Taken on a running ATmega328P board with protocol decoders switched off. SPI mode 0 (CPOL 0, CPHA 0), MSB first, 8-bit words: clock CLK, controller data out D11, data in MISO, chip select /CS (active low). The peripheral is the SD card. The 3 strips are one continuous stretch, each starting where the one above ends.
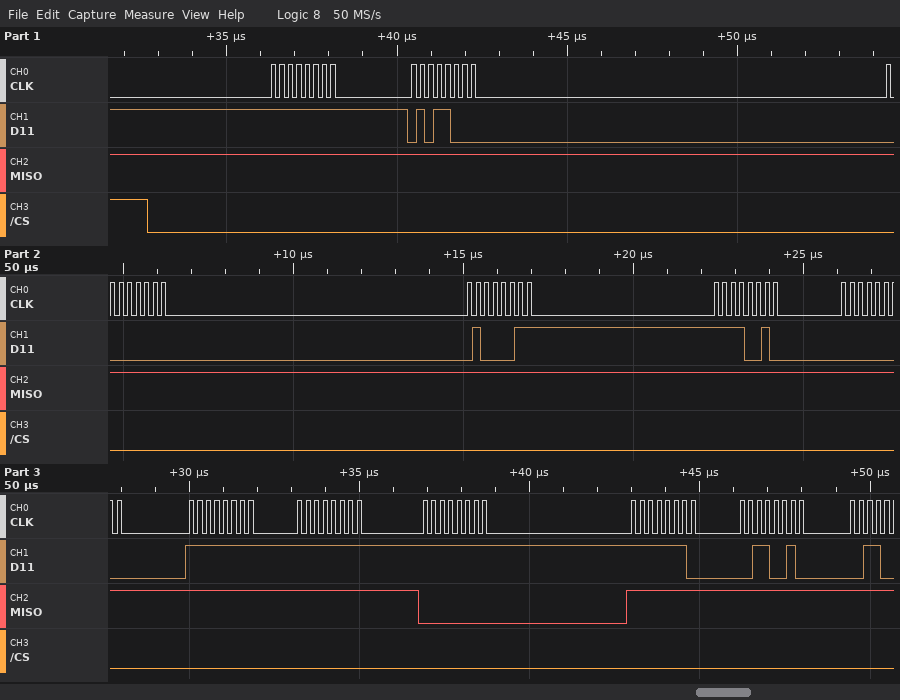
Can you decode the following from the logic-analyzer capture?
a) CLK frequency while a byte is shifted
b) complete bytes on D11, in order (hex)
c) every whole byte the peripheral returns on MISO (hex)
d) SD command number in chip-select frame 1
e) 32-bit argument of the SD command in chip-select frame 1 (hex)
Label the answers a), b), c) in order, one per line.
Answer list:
a) 4 MHz
b) FF 58 00 43 F2 00 FF FF FF FE 32
c) FF FF FF FF FF FF FF FF 00 FF FF
d) CMD24
e) 0x0043F200
